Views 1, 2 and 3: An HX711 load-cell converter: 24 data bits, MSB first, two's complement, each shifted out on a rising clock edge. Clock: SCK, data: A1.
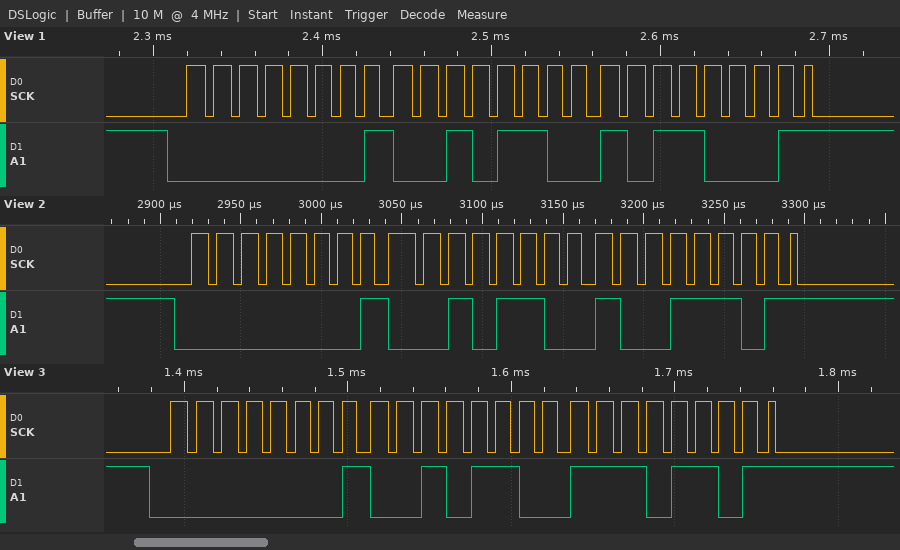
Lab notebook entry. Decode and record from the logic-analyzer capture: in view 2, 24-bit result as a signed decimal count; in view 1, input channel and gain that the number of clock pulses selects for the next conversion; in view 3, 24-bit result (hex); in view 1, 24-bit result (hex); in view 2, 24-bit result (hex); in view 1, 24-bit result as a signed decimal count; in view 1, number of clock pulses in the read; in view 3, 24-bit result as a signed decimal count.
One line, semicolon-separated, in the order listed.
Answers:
76957; channel A, gain 128; 0x012CED; 0x012CB1; 0x012C9D; 76977; 25; 77037
